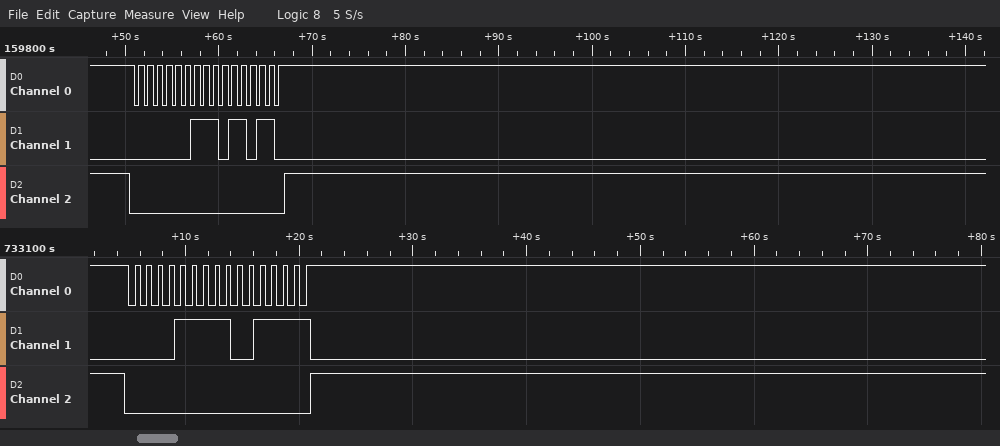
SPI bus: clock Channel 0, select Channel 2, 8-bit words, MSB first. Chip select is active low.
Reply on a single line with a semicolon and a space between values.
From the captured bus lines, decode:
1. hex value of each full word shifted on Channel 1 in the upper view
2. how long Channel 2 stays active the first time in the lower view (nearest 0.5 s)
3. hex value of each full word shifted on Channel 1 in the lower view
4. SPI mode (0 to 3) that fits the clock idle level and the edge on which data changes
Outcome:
03, B6; 16.5 s; 0F, 9F; 3
